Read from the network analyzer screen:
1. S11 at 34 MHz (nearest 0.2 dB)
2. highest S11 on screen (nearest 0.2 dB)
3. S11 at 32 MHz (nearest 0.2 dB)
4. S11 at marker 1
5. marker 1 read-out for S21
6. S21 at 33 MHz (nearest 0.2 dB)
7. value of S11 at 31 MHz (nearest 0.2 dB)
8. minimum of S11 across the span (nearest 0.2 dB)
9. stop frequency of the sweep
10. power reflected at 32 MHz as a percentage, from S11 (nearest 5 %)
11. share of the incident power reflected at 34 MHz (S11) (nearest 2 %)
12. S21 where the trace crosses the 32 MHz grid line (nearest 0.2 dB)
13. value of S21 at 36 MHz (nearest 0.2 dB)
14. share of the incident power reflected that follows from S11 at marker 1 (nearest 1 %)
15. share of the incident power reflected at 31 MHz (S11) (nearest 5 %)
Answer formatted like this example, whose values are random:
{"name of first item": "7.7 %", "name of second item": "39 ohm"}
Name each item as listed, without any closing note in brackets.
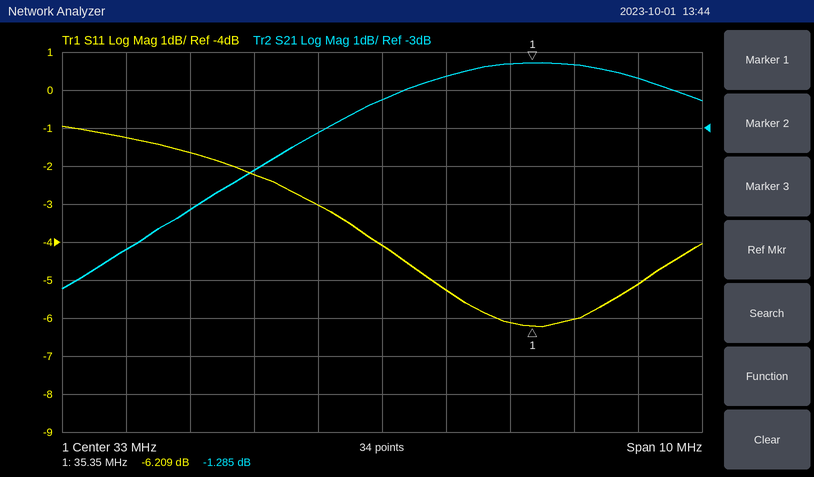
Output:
{"S11 at 34 MHz": "-5.2 dB", "highest S11 on screen": "-1.0 dB", "S11 at 32 MHz": "-3.0 dB", "S11 at marker 1": "-6.209 dB", "marker 1 read-out for S21": "-1.285 dB", "S21 at 33 MHz": "-2.2 dB", "value of S11 at 31 MHz": "-2.2 dB", "minimum of S11 across the span": "-6.2 dB", "stop frequency of the sweep": "38 MHz", "power reflected at 32 MHz as a percentage, from S11": "50 %", "share of the incident power reflected at 34 MHz (S11)": "30 %", "S21 where the trace crosses the 32 MHz grid line": "-3.2 dB", "value of S21 at 36 MHz": "-1.4 dB", "share of the incident power reflected that follows from S11 at marker 1": "24 %", "share of the incident power reflected at 31 MHz (S11)": "60 %"}
